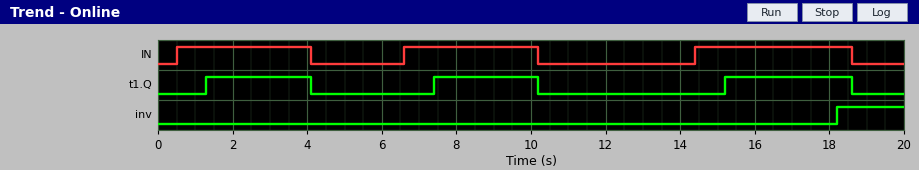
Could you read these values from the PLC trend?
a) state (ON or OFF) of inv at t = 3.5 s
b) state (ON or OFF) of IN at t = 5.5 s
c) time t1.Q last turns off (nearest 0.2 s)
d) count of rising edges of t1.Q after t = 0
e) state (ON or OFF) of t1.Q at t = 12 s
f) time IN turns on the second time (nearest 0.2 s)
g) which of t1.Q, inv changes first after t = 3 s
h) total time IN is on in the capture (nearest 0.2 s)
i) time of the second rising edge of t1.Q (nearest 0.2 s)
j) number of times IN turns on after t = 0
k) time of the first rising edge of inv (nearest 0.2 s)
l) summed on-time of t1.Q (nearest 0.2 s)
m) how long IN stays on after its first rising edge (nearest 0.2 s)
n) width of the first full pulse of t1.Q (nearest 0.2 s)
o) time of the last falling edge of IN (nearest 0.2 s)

OFF
OFF
18.6 s
3
OFF
6.6 s
t1.Q
11.4 s
7.4 s
3
18.2 s
9.0 s
3.6 s
2.8 s
18.6 s
